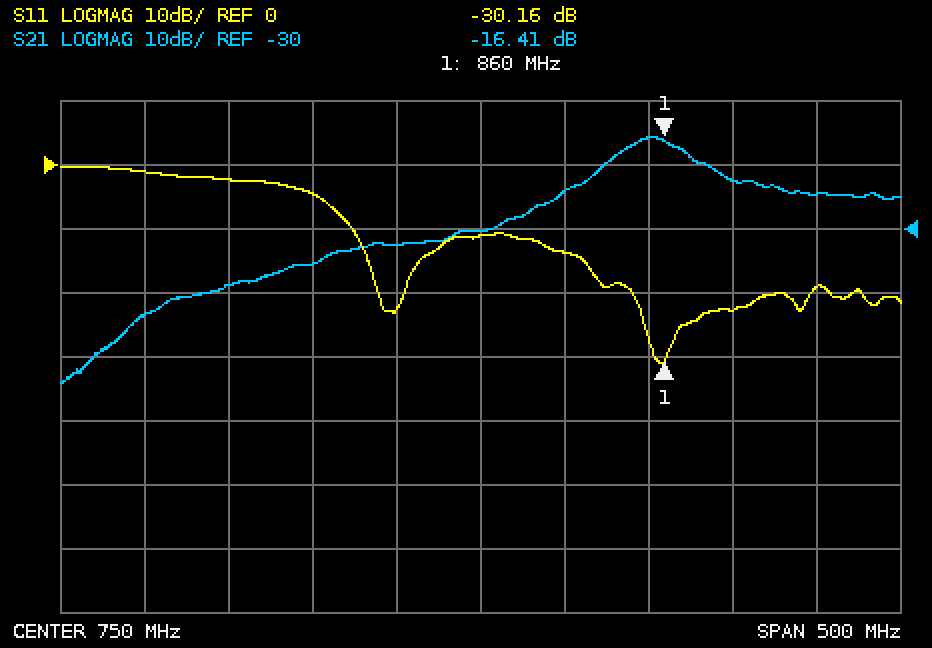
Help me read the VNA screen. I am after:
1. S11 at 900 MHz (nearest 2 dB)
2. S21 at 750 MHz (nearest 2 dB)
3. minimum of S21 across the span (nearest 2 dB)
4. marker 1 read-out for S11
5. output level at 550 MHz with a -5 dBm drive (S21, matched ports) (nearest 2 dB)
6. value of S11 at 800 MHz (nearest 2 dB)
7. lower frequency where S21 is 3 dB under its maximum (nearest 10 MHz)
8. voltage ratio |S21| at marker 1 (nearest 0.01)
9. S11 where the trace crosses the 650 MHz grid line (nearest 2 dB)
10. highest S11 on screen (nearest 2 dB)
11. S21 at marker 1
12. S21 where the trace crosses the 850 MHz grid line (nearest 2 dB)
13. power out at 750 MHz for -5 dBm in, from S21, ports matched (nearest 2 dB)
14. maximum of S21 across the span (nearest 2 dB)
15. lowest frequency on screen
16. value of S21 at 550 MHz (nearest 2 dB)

-22 dB
-30 dB
-54 dB
-30.16 dB
-48 dBm
-14 dB
830 MHz
0.15
-4 dB
0 dB
-16.41 dB
-16 dB
-36 dBm
-16 dB
500 MHz
-44 dB
